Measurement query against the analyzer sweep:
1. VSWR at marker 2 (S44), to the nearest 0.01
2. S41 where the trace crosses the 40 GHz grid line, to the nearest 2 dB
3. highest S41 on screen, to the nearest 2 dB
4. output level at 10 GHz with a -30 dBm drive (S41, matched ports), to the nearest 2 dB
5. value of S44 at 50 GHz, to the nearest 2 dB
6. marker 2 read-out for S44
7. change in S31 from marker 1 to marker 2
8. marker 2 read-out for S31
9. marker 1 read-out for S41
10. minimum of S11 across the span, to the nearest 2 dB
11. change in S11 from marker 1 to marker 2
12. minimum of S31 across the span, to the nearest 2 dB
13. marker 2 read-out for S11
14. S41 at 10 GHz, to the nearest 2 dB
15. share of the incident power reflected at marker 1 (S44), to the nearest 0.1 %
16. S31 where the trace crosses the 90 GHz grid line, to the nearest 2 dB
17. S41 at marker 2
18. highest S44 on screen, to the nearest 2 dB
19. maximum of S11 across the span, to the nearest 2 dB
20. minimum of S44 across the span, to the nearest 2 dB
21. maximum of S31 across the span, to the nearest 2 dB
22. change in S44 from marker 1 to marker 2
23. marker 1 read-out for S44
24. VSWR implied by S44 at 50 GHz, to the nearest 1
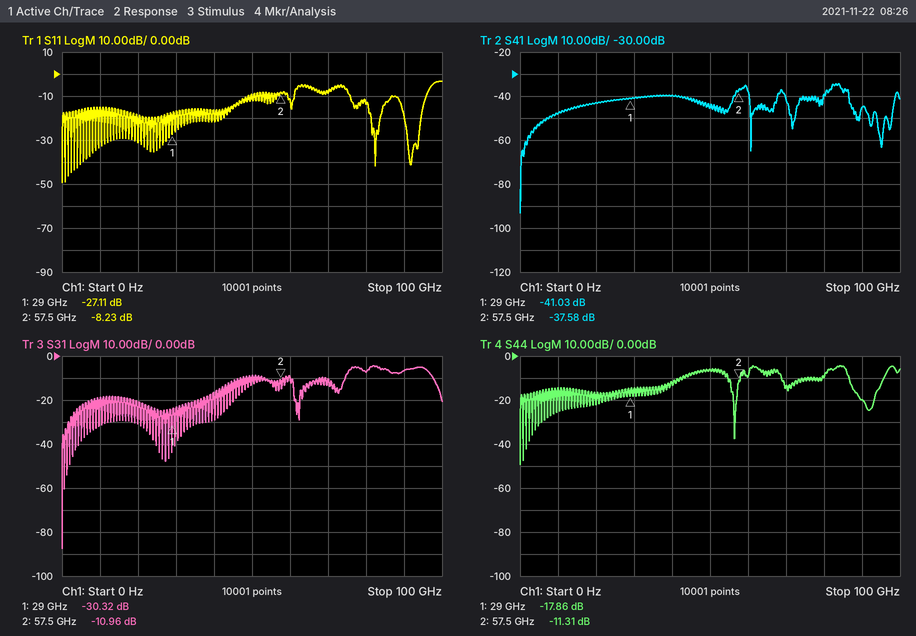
1.75
-40 dB
-34 dB
-78 dBm
-6 dB
-11.31 dB
19.36 dB
-10.96 dB
-41.03 dB
-50 dB
18.88 dB
-88 dB
-8.23 dB
-48 dB
1.6 %
-6 dB
-37.58 dB
-4 dB
-4 dB
-50 dB
-4 dB
6.55 dB
-17.86 dB
3
